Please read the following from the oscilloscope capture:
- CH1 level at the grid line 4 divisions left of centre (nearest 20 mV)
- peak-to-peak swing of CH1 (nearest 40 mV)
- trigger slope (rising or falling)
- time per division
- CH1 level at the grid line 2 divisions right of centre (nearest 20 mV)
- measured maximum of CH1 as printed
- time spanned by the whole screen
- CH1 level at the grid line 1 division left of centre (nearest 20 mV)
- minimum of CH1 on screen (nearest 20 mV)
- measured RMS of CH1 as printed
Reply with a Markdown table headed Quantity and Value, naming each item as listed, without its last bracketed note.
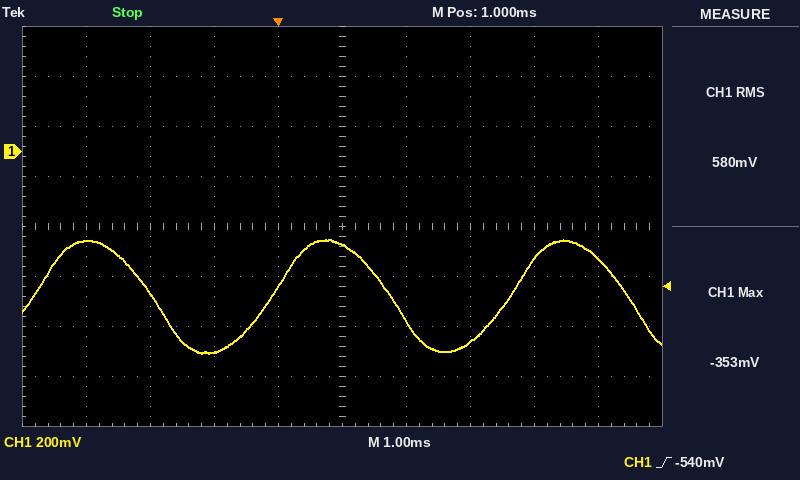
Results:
| Quantity | Value |
|---|---|
| CH1 level at the grid line 4 divisions left of centre | -360 mV |
| peak-to-peak swing of CH1 | 440 mV |
| trigger slope | rising |
| time per division | 1 ms |
| CH1 level at the grid line 2 divisions right of centre | -760 mV |
| measured maximum of CH1 as printed | -353 mV |
| time spanned by the whole screen | 10 ms |
| CH1 level at the grid line 1 division left of centre | -540 mV |
| minimum of CH1 on screen | -800 mV |
| measured RMS of CH1 as printed | 580 mV |
